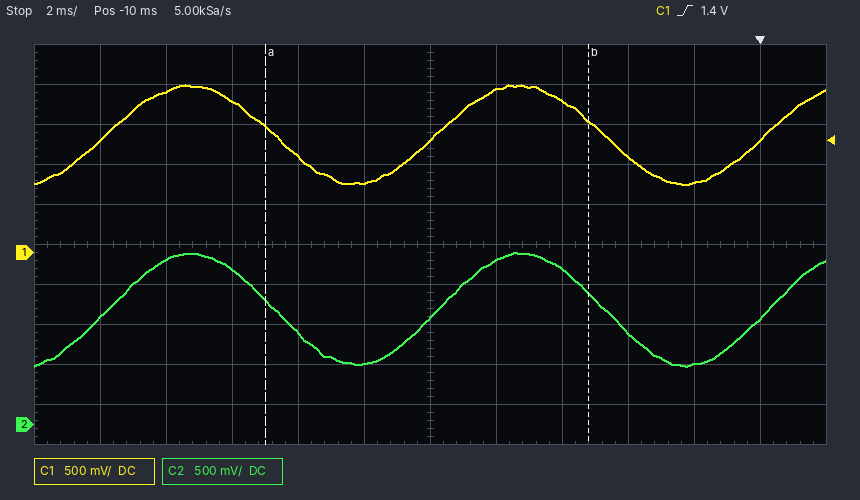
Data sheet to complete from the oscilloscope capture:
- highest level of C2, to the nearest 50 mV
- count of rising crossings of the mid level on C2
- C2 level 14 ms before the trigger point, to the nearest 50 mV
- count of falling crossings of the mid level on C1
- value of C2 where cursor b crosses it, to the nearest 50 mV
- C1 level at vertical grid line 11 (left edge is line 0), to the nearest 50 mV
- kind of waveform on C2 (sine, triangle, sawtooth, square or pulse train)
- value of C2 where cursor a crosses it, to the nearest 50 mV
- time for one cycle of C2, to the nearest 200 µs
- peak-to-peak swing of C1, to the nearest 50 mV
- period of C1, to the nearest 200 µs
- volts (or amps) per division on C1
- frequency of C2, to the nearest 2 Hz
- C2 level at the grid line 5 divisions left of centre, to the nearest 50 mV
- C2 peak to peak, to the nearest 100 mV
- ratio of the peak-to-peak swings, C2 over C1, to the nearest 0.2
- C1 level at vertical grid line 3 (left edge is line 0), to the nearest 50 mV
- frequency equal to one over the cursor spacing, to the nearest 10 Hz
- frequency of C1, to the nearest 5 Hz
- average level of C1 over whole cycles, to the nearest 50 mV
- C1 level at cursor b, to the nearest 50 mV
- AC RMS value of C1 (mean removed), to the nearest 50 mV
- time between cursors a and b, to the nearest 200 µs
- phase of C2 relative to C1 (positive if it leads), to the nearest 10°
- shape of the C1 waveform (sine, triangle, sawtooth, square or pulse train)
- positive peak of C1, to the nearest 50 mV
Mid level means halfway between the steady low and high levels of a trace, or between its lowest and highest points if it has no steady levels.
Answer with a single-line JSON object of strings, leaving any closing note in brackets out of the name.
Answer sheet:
{"highest level of C2, to the nearest 50 mV": "2.15 V", "count of rising crossings of the mid level on C2": "3", "C2 level 14 ms before the trigger point, to the nearest 50 mV": "1.15 V", "count of falling crossings of the mid level on C1": "2", "value of C2 where cursor b crosses it, to the nearest 50 mV": "1.65 V", "C1 level at vertical grid line 11 (left edge is line 0), to the nearest 50 mV": "1.40 V", "kind of waveform on C2": "sine", "value of C2 where cursor a crosses it, to the nearest 50 mV": "1.55 V", "time for one cycle of C2, to the nearest 200 µs": "10.0 ms", "peak-to-peak swing of C1, to the nearest 50 mV": "1.25 V", "period of C1, to the nearest 200 µs": "10.0 ms", "volts (or amps) per division on C1": "500 mV", "frequency of C2, to the nearest 2 Hz": "100 Hz", "C2 level at the grid line 5 divisions left of centre, to the nearest 50 mV": "1.35 V", "C2 peak to peak, to the nearest 100 mV": "1.40 V", "ratio of the peak-to-peak swings, C2 over C1, to the nearest 0.2": "1.2", "C1 level at vertical grid line 3 (left edge is line 0), to the nearest 50 mV": "1.90 V", "frequency equal to one over the cursor spacing, to the nearest 10 Hz": "100 Hz", "frequency of C1, to the nearest 5 Hz": "100 Hz", "average level of C1 over whole cycles, to the nearest 50 mV": "1.50 V", "C1 level at cursor b, to the nearest 50 mV": "1.65 V", "AC RMS value of C1 (mean removed), to the nearest 50 mV": "450 mV", "time between cursors a and b, to the nearest 200 µs": "9.8 ms", "phase of C2 relative to C1 (positive if it leads), to the nearest 10°": "0°", "shape of the C1 waveform": "sine", "positive peak of C1, to the nearest 50 mV": "2.10 V"}
